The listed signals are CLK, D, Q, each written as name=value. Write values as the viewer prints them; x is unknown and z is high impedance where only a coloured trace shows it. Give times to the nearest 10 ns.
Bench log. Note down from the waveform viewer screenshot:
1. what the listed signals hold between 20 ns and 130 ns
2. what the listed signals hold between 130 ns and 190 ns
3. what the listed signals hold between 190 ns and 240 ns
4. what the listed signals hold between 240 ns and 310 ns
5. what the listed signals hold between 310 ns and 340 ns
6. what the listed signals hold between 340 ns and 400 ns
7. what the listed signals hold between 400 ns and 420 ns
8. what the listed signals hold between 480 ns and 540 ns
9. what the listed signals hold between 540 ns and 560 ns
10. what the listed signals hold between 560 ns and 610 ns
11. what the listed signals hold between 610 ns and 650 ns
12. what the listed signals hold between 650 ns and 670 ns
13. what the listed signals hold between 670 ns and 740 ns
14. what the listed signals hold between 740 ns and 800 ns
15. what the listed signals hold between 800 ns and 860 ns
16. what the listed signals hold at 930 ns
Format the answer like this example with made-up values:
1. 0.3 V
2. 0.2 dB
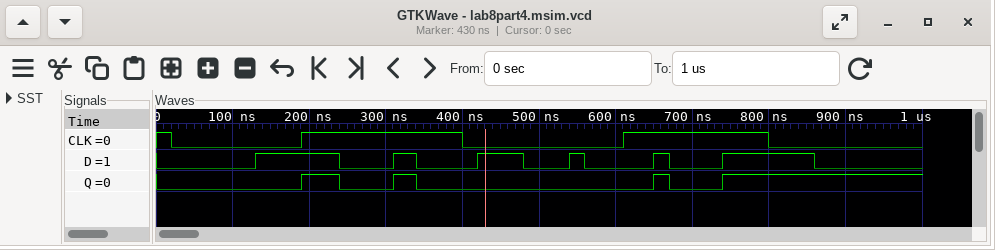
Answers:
1. CLK=0, D=0, Q=0
2. CLK=0, D=1, Q=0
3. CLK=1, D=1, Q=1
4. CLK=1, D=0, Q=0
5. CLK=1, D=1, Q=1
6. CLK=1, D=0, Q=0
7. CLK=0, D=0, Q=0
8. CLK=0, D=0, Q=0
9. CLK=0, D=1, Q=0
10. CLK=0, D=0, Q=0
11. CLK=1, D=0, Q=0
12. CLK=1, D=1, Q=1
13. CLK=1, D=0, Q=0
14. CLK=1, D=1, Q=1
15. CLK=0, D=1, Q=1
16. CLK=0, D=0, Q=1
